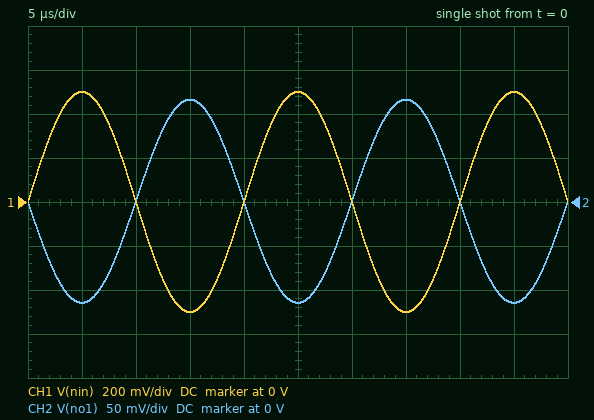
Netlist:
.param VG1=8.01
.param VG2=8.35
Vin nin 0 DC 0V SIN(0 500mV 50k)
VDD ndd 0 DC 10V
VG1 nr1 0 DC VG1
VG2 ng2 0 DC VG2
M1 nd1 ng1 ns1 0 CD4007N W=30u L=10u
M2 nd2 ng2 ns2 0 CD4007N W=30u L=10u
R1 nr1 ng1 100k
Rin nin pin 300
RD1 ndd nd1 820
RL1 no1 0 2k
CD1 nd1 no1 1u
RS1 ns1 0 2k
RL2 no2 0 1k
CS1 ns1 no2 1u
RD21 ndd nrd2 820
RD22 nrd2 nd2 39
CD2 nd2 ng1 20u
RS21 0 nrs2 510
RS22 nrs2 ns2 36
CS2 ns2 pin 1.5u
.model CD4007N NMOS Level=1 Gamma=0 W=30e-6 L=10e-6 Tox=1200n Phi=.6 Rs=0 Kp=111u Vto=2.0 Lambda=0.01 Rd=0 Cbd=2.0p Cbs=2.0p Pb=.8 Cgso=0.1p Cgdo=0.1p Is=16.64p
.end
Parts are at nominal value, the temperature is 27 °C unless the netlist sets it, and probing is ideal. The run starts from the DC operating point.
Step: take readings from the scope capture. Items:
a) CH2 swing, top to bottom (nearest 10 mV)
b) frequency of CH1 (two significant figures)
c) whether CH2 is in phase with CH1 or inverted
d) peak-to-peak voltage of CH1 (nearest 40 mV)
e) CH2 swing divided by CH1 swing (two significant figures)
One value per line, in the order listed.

230 mV
50 kHz
inverted
1.00 V
0.23
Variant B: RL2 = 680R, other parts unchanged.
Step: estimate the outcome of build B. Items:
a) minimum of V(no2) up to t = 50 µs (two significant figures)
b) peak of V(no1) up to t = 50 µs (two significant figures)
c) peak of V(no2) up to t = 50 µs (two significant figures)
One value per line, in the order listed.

-110 mV
130 mV
110 mV
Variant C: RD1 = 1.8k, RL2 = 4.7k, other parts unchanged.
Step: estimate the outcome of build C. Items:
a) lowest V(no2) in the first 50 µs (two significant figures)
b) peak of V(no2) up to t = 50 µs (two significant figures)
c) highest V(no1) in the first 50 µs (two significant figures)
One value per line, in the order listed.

-190 mV
190 mV
130 mV
